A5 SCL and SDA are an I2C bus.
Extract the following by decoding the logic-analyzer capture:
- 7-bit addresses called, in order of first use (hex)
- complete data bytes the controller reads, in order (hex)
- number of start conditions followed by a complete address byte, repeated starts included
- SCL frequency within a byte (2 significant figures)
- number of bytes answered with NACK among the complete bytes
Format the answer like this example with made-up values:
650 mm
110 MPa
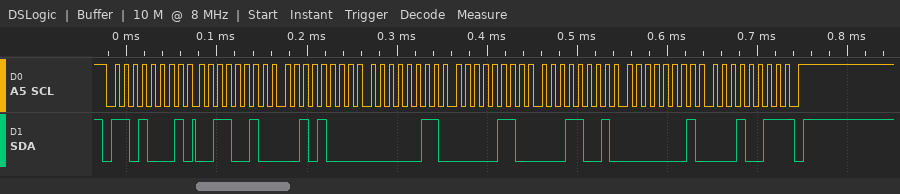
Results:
0x68
32 28 03 06 19 01 13
1
100 kHz
1
